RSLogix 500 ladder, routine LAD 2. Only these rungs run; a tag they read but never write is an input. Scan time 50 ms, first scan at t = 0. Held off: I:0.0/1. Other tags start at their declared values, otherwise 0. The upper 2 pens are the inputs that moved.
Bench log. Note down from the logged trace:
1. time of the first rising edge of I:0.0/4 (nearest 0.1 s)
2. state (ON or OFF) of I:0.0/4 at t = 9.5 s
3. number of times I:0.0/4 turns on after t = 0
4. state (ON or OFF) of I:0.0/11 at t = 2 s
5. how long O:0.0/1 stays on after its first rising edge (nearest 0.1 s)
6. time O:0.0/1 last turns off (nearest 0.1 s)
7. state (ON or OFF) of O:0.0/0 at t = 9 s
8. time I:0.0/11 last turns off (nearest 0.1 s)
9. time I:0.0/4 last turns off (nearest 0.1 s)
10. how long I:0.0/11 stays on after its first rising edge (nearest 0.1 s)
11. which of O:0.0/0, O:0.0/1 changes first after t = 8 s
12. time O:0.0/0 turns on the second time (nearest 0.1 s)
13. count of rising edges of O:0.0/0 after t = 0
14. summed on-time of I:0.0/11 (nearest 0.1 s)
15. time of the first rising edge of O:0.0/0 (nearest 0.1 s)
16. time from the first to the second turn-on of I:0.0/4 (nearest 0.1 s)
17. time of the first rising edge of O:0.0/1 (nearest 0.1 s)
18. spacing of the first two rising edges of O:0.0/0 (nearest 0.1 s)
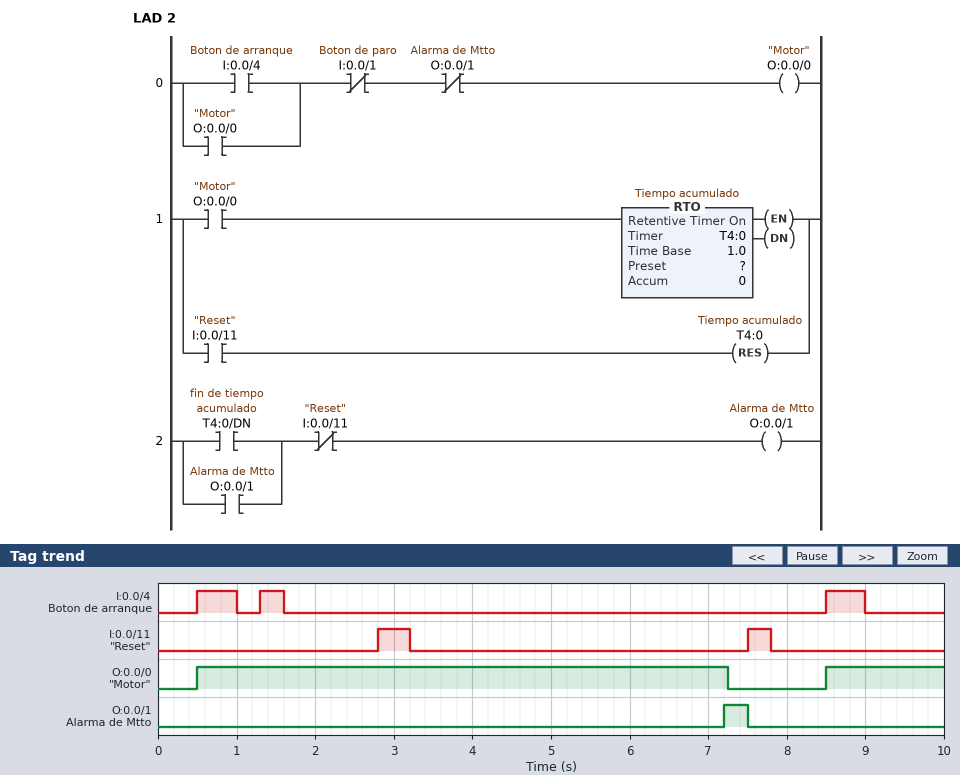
0.5 s
OFF
3
OFF
0.3 s
7.5 s
ON
7.8 s
9.0 s
0.4 s
O:0.0/0
8.5 s
2
0.7 s
0.5 s
0.8 s
7.2 s
8.0 s
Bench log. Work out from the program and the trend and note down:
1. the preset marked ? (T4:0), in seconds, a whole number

4 s
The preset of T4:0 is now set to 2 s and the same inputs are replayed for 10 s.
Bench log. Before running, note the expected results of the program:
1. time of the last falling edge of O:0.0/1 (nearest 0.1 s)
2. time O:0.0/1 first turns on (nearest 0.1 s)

2.8 s
2.5 s
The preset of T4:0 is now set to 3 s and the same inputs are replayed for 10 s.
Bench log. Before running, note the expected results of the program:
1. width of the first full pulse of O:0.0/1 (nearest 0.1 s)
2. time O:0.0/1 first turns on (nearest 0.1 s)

1.3 s
6.2 s
